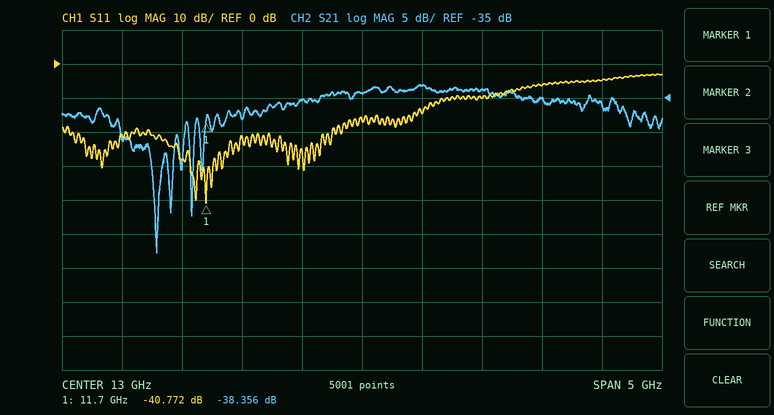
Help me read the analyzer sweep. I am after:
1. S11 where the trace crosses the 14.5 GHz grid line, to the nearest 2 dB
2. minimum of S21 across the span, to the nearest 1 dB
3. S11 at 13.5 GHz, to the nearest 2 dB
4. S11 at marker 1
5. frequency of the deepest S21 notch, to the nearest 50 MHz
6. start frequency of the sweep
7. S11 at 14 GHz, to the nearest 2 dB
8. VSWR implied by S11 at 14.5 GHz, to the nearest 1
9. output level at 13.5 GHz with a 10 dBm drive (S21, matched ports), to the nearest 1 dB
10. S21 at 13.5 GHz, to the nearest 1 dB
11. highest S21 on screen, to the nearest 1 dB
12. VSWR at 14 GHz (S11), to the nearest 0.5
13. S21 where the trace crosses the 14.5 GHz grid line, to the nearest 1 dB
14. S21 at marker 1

-6 dB
-58 dB
-14 dB
-40.772 dB
11.30 GHz
10.5 GHz
-10 dB
3
-23 dBm
-33 dB
-33 dB
2.0
-35 dB
-38.356 dB
